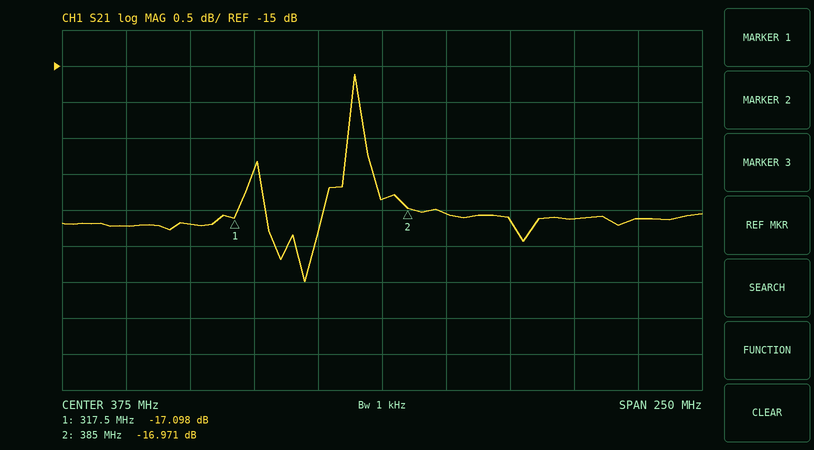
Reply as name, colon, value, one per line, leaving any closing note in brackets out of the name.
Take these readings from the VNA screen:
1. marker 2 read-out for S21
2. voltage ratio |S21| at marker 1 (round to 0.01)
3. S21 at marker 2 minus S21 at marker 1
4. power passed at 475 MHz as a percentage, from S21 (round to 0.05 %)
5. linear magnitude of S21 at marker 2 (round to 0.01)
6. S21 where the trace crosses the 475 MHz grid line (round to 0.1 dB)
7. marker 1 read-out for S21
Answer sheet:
marker 2 read-out for S21: -16.971 dB
voltage ratio |S21| at marker 1: 0.14
S21 at marker 2 minus S21 at marker 1: 0.127 dB
power passed at 475 MHz as a percentage, from S21: 1.95 %
linear magnitude of S21 at marker 2: 0.14
S21 where the trace crosses the 475 MHz grid line: -17.1 dB
marker 1 read-out for S21: -17.098 dB
